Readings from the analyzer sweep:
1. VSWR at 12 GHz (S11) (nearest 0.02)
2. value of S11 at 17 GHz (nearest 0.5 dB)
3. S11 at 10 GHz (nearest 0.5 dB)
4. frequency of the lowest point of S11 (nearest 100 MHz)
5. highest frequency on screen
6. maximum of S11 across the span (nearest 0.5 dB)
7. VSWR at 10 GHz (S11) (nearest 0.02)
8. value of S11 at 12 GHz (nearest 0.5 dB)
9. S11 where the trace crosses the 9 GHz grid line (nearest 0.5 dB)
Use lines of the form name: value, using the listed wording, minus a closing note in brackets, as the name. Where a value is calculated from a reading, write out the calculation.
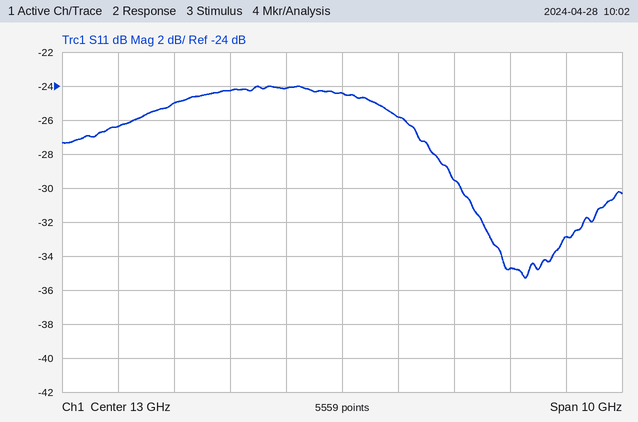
VSWR at 12 GHz (S11): |Γ| = 10^(-24/20) = 0.0631; VSWR = (1 + 0.0631)/(1 − 0.0631) ≈ 1.13, so 1.14 to the nearest 0.02
value of S11 at 17 GHz: -33.0 dB
S11 at 10 GHz: -25.0 dB
frequency of the lowest point of S11: 16.3 GHz
highest frequency on screen: 18 GHz
maximum of S11 across the span: -24.0 dB
VSWR at 10 GHz (S11): |Γ| = 10^(-25/20) = 0.0562; VSWR = (1 + 0.0562)/(1 − 0.0562) ≈ 1.12
value of S11 at 12 GHz: -24.0 dB
S11 where the trace crosses the 9 GHz grid line: -26.5 dB
